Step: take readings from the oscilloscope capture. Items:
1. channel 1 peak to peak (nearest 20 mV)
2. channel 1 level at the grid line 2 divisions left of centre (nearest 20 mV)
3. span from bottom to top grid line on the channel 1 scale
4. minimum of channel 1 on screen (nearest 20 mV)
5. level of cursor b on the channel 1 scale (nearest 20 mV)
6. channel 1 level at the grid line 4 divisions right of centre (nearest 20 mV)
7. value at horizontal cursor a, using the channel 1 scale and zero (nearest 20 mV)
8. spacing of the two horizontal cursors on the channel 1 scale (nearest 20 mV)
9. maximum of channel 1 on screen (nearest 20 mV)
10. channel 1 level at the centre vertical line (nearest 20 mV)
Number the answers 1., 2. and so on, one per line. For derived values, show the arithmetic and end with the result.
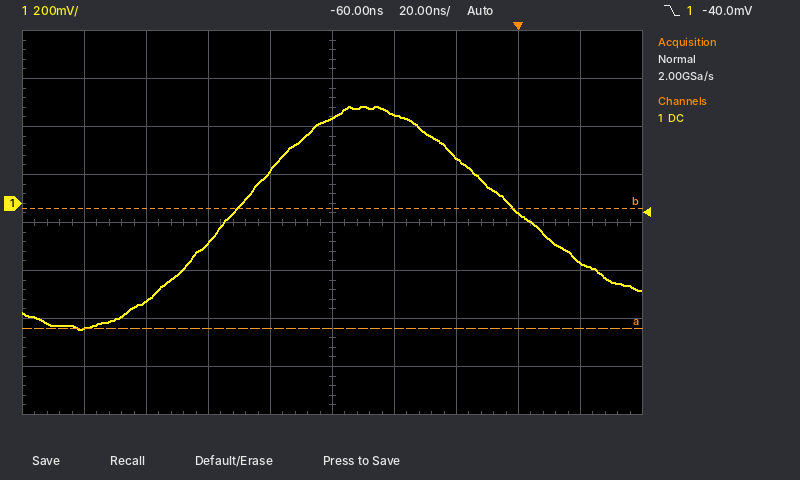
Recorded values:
1. 400 mV − (-520 mV) = 920 mV
2. -160 mV
3. 1.6 V
4. -520 mV
5. -20 mV
6. -240 mV
7. -520 mV
8. 500 mV
9. 400 mV
10. 360 mV
